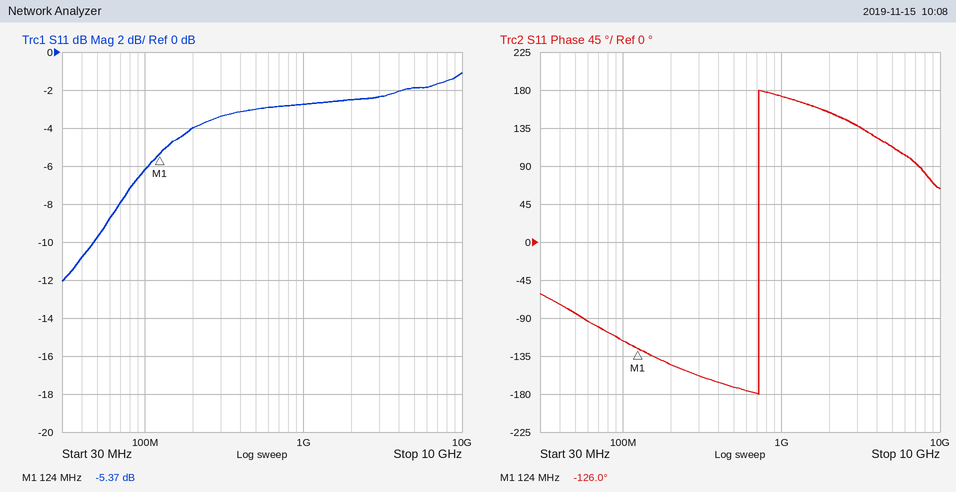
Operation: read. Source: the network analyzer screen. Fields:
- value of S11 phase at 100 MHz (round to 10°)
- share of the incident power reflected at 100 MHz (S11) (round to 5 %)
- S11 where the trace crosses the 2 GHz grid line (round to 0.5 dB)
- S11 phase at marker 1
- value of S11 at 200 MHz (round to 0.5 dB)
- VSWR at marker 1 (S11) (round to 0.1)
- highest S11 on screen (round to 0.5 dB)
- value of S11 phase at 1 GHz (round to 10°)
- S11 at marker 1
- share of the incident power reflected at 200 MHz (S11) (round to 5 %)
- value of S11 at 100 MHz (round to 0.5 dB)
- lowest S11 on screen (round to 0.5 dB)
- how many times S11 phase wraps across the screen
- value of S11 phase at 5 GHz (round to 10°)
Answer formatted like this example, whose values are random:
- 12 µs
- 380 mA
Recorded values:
- -120°
- 25 %
- -2.5 dB
- -126.0°
- -4.0 dB
- 3.3
- -1.0 dB
- 170°
- -5.37 dB
- 40 %
- -6.0 dB
- -12.0 dB
- 1
- 110°
